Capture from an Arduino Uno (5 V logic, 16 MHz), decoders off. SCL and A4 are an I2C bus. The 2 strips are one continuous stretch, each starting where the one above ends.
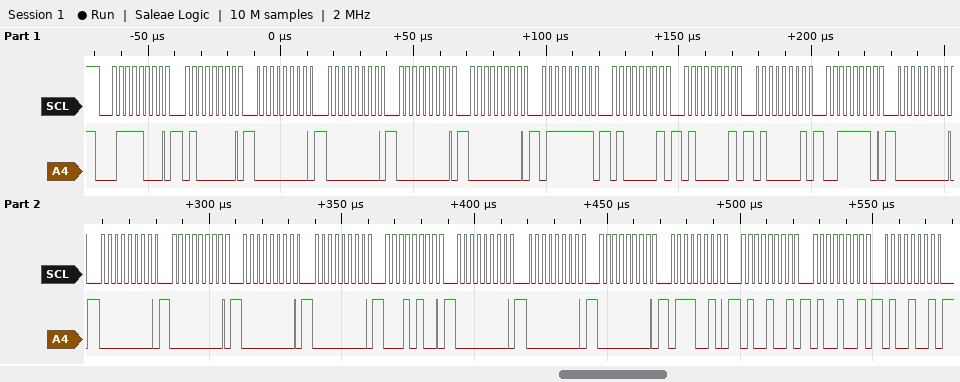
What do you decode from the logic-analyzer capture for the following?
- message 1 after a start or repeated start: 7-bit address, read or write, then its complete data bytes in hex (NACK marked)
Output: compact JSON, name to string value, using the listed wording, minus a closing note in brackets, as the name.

{"message 1 after a start or repeated start: 7-bit address, read or write, then its complete data bytes in hex": "0x3C write: 40 00 00 00 00 7F 41 41 41 3E 00 00 00 00 00 14 00 00 00 72 49 49 49"}
